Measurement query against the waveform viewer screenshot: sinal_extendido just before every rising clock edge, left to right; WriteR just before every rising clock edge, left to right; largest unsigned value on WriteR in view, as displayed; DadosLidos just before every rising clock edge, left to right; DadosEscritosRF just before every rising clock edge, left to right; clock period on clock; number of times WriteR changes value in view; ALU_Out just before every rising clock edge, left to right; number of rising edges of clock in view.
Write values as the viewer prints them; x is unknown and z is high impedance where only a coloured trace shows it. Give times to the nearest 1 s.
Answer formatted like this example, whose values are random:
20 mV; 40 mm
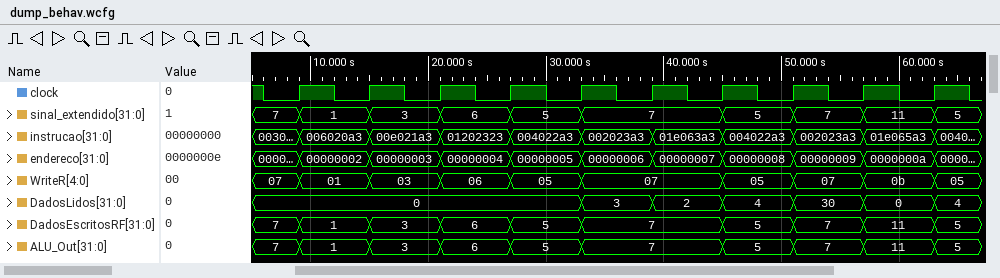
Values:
7, 1, 3, 6, 5, 7, 7, 5, 7, 11; 07, 01, 03, 06, 05, 07, 07, 05, 07, 0b; 0b; 0, 0, 0, 0, 0, 3, 2, 4, 30, 0; 7, 1, 3, 6, 5, 7, 7, 5, 7, 11; 6 s; 9; 7, 1, 3, 6, 5, 7, 7, 5, 7, 11; 10
